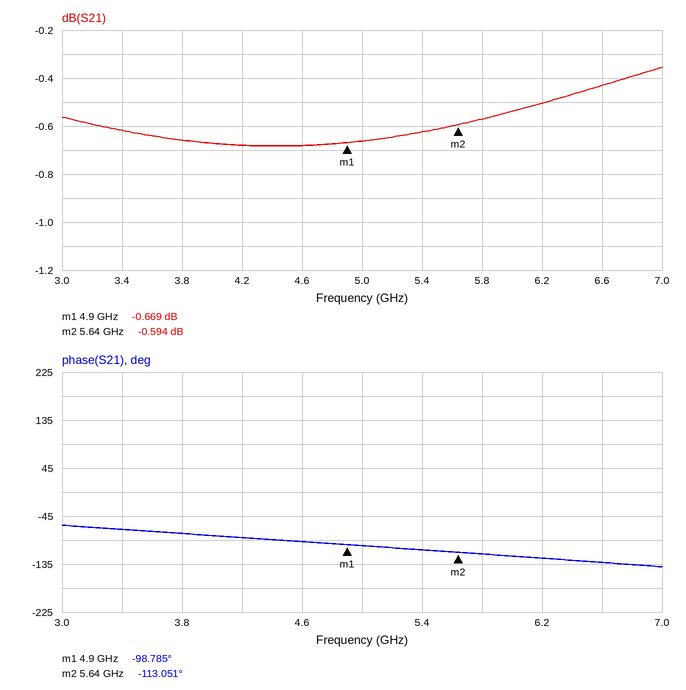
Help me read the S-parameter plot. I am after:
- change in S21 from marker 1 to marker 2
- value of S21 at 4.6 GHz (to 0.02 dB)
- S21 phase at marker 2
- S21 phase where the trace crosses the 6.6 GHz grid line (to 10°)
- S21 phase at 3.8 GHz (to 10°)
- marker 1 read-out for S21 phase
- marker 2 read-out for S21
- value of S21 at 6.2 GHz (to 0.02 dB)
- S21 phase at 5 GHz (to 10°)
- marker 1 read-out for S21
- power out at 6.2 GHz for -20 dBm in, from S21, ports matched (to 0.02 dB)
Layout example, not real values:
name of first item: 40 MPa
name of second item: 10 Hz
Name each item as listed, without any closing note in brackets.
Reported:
change in S21 from marker 1 to marker 2: 0.075 dB
value of S21 at 4.6 GHz: -0.68 dB
S21 phase at marker 2: -113.051°
S21 phase where the trace crosses the 6.6 GHz grid line: -130°
S21 phase at 3.8 GHz: -80°
marker 1 read-out for S21 phase: -98.785°
marker 2 read-out for S21: -0.594 dB
value of S21 at 6.2 GHz: -0.50 dB
S21 phase at 5 GHz: -100°
marker 1 read-out for S21: -0.669 dB
power out at 6.2 GHz for -20 dBm in, from S21, ports matched: -20.50 dBm
